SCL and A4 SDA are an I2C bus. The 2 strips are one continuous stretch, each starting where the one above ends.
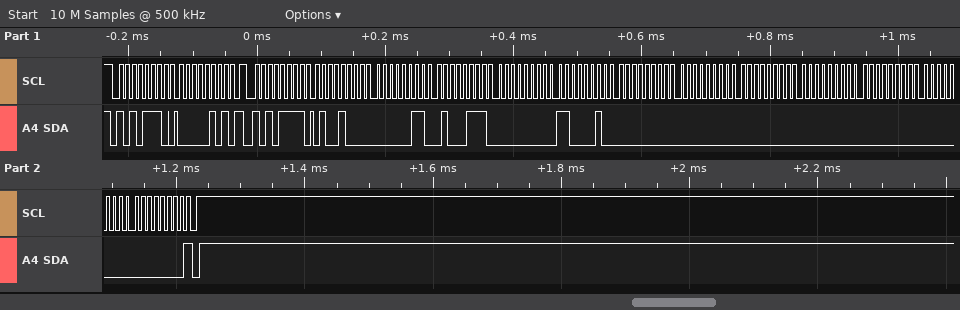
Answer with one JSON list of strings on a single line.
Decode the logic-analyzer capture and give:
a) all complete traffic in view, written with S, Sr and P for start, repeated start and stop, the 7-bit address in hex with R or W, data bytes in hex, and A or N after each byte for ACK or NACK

["S 57W A 05 A Sr 57R A 48 A 03 A 47 A 00 A C2 A 00 A 00 A 00 A 00 A 00 A 00 A 00 N P"]
